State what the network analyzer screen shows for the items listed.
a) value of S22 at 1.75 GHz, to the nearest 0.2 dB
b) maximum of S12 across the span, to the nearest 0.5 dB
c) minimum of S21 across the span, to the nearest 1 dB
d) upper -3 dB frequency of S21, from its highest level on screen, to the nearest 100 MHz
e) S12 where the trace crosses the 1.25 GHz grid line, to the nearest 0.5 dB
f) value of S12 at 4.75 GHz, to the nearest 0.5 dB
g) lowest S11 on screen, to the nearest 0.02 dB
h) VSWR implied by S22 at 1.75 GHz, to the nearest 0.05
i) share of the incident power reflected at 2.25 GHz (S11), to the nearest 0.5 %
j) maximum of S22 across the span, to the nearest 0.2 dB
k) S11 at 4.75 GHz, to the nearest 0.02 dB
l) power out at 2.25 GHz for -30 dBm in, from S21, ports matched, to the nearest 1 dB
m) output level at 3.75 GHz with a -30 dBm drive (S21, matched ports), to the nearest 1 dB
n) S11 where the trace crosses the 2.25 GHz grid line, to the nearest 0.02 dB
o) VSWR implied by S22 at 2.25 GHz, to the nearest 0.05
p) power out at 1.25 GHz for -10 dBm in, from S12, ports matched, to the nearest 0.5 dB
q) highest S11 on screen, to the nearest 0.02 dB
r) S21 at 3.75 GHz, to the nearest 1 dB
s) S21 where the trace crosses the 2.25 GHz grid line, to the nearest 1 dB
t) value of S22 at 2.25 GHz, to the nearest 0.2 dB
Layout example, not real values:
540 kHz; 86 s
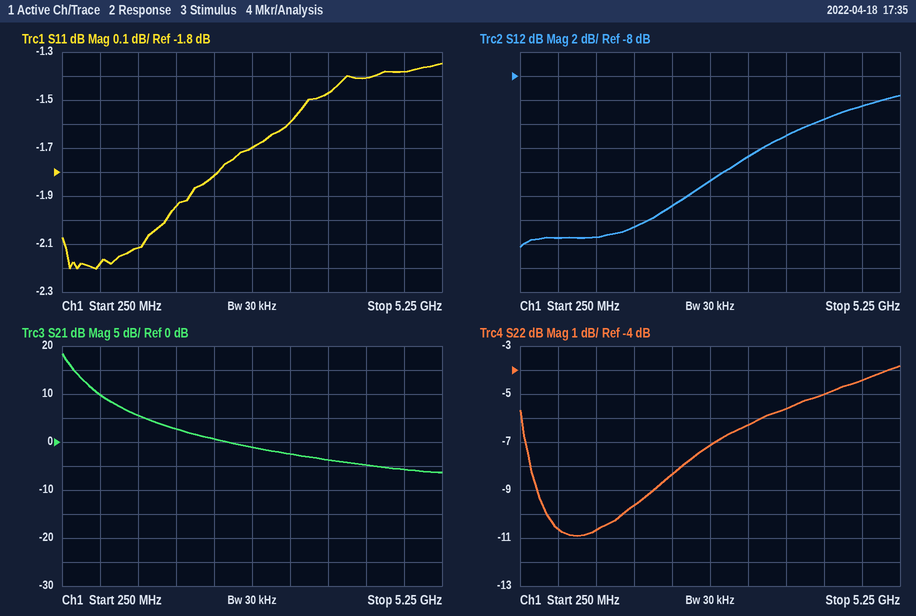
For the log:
-9.6 dB; -9.5 dB; -6 dB; 400 MHz; -21.5 dB; -10.5 dB; -2.20 dB; 2.00; 66.0 %; -3.8 dB; -1.38 dB; -29 dBm; -34 dBm; -1.82 dB; 2.25; -31.5 dBm; -1.34 dB; -4 dB; 1 dB; -8.4 dB
